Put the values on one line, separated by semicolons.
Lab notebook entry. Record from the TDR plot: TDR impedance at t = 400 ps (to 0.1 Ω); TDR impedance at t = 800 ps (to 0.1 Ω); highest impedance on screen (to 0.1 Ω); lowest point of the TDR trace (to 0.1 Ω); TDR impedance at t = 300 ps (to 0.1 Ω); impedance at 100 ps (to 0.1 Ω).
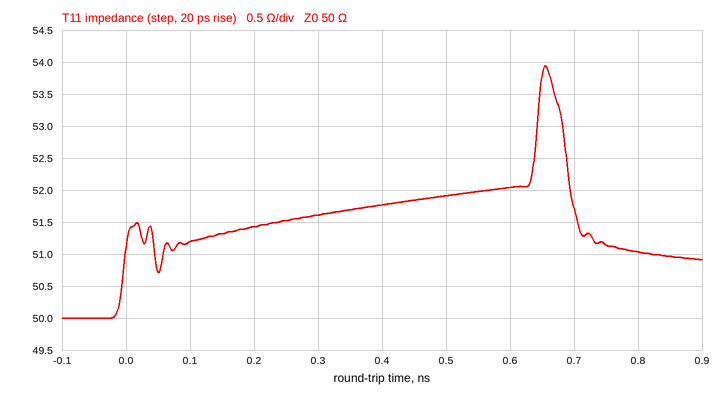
51.8 Ω; 51.0 Ω; 53.9 Ω; 50.0 Ω; 51.6 Ω; 51.2 Ω
